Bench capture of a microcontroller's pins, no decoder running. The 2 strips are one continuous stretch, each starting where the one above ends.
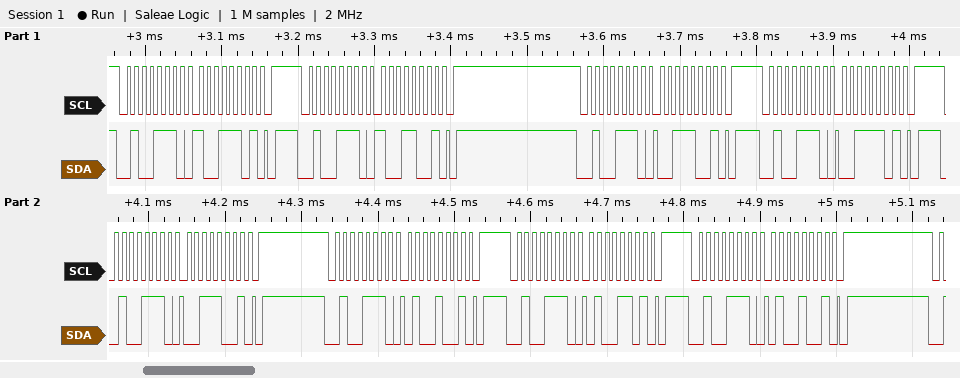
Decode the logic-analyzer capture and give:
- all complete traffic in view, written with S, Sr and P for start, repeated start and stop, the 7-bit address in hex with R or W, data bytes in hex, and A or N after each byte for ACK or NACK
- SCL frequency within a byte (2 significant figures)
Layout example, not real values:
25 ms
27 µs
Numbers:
S 27W A 9D A P S 27W A 99 A P S 27W A 39 A P S 27W A 3D A P S 27W A 39 A P S 27W A 49 A P S 27W A 4D A P S 27W A 49 A P
100 kHz
